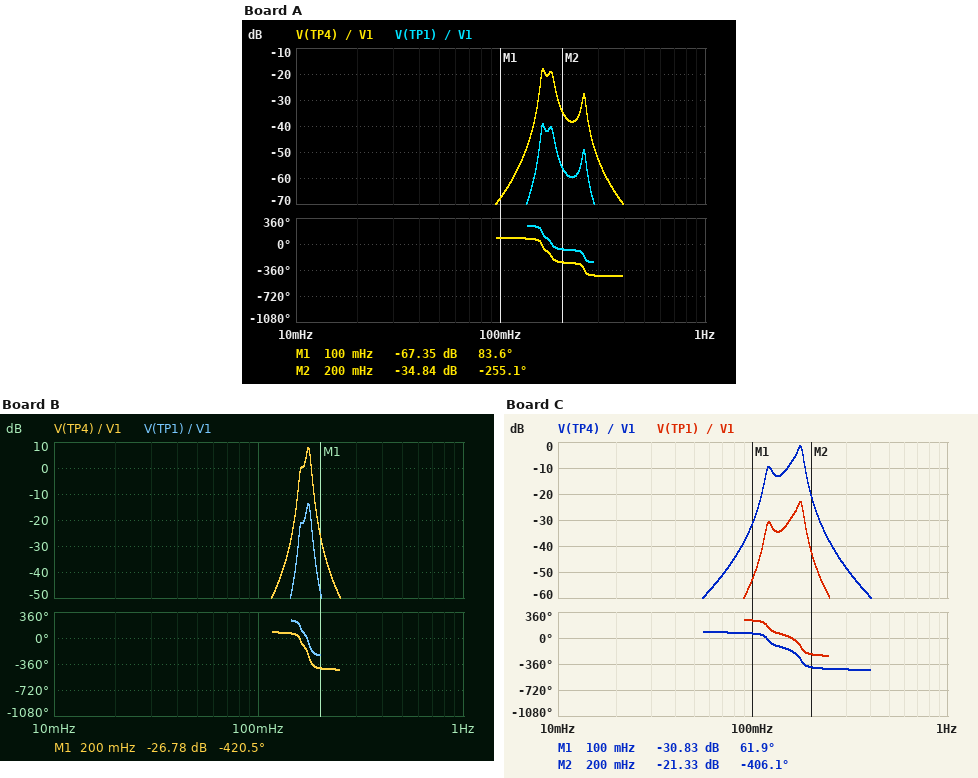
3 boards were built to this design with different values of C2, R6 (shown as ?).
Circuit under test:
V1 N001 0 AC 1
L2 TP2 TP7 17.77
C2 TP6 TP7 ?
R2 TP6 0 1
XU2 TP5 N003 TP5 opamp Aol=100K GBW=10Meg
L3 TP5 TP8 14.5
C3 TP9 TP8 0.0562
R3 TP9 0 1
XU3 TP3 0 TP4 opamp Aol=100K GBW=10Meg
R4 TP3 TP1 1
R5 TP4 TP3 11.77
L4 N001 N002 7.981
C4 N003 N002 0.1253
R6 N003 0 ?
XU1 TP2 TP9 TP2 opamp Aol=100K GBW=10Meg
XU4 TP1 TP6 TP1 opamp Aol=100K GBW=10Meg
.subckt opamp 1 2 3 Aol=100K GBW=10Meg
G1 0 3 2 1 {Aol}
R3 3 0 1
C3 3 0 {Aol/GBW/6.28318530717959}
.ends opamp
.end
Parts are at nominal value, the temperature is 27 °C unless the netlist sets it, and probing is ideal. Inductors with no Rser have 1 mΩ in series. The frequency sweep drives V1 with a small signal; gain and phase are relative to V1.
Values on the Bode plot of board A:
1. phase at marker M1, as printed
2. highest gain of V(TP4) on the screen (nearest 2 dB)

83.6 deg
-18 dB
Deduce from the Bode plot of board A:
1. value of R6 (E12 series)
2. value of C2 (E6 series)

0.33 Ω
22 mF
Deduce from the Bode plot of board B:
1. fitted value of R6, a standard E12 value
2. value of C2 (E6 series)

0.33 Ω
47 mF
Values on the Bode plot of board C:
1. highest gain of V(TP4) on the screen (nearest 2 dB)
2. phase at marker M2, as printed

-2 dB
-406.1 deg
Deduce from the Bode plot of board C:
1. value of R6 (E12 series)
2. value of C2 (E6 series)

1.8 Ω
100 mF
